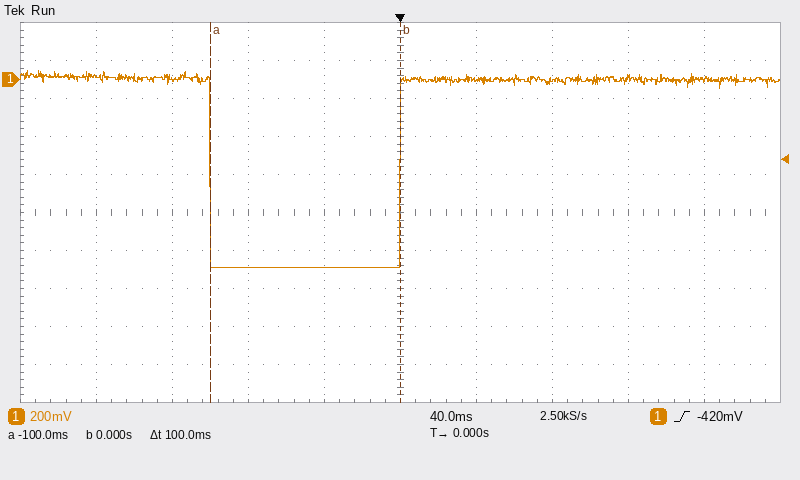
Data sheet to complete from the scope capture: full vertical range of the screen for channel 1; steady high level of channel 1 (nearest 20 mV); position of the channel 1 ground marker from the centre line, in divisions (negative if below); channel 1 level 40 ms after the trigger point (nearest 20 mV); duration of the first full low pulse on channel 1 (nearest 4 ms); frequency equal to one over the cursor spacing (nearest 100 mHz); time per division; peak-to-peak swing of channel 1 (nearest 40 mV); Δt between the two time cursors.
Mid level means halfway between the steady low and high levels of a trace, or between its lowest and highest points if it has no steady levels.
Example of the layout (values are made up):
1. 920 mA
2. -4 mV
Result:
1. 2 V
2. 0 mV
3. +3.5 div
4. 0 mV
5. 100 ms
6. 10.0 Hz
7. 40 ms
8. 1.04 V
9. 100 ms
